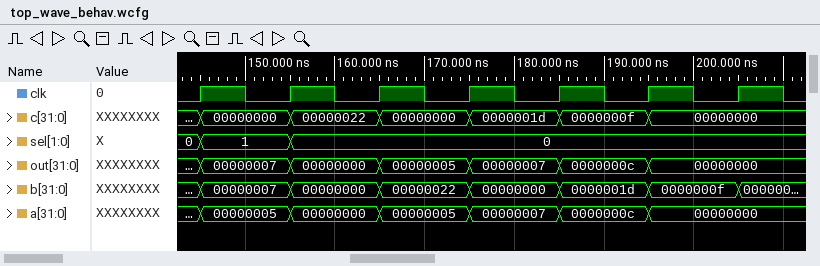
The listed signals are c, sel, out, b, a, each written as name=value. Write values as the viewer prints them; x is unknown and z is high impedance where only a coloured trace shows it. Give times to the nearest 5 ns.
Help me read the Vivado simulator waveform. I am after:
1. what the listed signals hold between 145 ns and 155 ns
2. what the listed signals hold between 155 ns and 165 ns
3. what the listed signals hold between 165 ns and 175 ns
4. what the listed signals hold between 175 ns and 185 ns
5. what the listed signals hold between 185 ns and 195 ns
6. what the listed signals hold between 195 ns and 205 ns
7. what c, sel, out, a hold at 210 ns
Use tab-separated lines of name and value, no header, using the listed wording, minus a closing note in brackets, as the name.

what the listed signals hold between 145 ns and 155 ns	c=00000000, sel=1, out=00000007, b=00000007, a=00000005
what the listed signals hold between 155 ns and 165 ns	c=00000022, sel=0, out=00000000, b=00000000, a=00000000
what the listed signals hold between 165 ns and 175 ns	c=00000000, sel=0, out=00000005, b=00000022, a=00000005
what the listed signals hold between 175 ns and 185 ns	c=0000001d, sel=0, out=00000007, b=00000000, a=00000007
what the listed signals hold between 185 ns and 195 ns	c=0000000f, sel=0, out=0000000c, b=0000001d, a=0000000c
what the listed signals hold between 195 ns and 205 ns	c=00000000, sel=0, out=00000000, b=0000000f, a=00000000
what c, sel, out, a hold at 210 ns	c=00000000, sel=0, out=00000000, a=00000000
